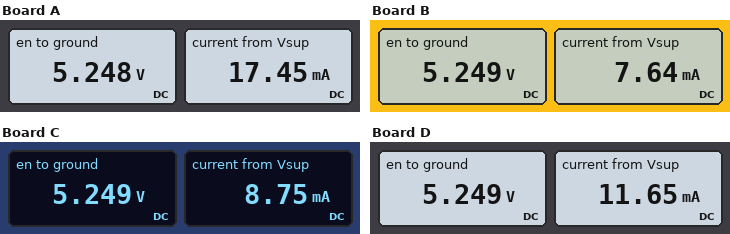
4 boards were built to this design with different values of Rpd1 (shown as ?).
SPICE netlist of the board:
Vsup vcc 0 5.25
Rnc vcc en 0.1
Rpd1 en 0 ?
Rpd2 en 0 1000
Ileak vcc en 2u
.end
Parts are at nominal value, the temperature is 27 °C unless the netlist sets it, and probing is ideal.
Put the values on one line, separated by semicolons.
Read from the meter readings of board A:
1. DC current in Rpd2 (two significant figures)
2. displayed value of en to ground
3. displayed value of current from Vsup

5.2 mA; 5.248 V; 17.45 mA
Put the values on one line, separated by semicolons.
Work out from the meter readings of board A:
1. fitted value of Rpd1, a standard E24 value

430 Ω
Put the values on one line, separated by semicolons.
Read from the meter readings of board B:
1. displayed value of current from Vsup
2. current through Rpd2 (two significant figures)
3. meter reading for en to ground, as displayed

7.64 mA; 5.2 mA; 5.249 V
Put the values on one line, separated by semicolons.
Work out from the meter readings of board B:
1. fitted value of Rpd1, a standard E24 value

2.2 kΩ
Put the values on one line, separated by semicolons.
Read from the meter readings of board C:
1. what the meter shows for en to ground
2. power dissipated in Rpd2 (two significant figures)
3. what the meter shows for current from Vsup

5.249 V; 28 mW; 8.75 mA
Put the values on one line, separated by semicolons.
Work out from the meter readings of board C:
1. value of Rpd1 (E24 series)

1.5 kΩ
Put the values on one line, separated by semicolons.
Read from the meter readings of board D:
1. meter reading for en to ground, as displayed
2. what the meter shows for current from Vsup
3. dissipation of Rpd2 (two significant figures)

5.249 V; 11.65 mA; 28 mW
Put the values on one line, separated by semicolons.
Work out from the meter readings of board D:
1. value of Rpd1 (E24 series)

820 Ω
